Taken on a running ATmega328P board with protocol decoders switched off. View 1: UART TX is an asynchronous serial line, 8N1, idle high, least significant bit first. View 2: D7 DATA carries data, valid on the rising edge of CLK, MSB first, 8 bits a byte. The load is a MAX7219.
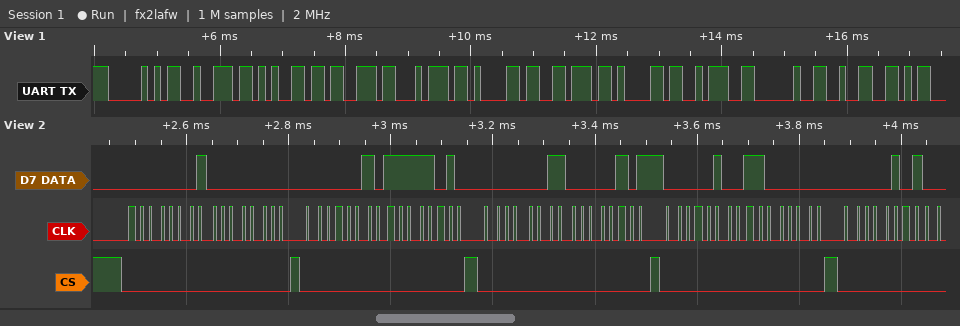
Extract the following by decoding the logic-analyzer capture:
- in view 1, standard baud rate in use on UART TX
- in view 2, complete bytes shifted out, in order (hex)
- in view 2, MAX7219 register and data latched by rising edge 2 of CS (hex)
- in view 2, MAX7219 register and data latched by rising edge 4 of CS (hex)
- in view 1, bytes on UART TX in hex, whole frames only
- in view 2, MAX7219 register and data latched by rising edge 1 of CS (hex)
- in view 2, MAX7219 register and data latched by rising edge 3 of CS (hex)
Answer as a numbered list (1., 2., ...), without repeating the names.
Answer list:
1. 9600 baud
2. 01 00 02 FA 03 05 04 C0 05
3. register 0x2, data 0xFA
4. register 0x4, data 0xC0
5. 50 72 65 73 74 61 76 61 3A 20 32
6. register 0x1, data 0x00
7. register 0x3, data 0x05
